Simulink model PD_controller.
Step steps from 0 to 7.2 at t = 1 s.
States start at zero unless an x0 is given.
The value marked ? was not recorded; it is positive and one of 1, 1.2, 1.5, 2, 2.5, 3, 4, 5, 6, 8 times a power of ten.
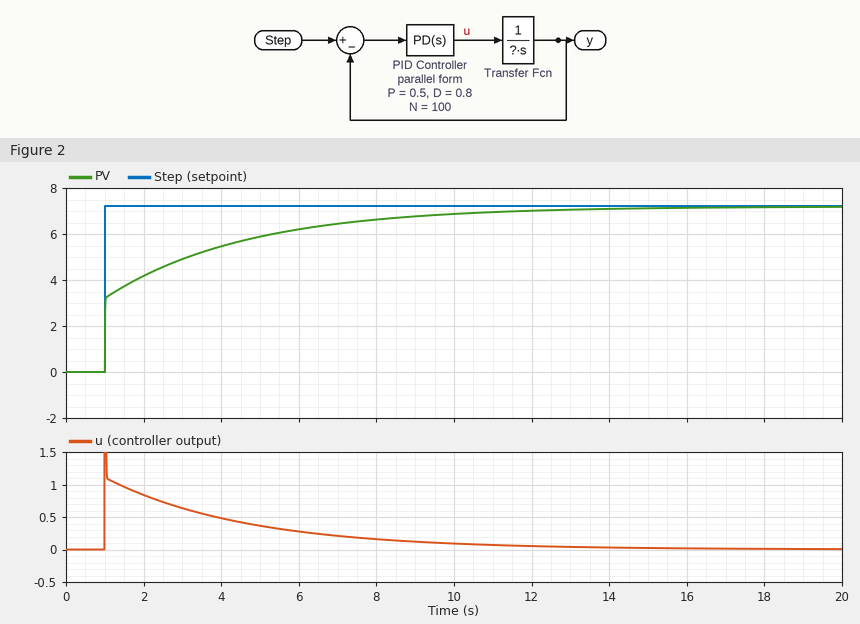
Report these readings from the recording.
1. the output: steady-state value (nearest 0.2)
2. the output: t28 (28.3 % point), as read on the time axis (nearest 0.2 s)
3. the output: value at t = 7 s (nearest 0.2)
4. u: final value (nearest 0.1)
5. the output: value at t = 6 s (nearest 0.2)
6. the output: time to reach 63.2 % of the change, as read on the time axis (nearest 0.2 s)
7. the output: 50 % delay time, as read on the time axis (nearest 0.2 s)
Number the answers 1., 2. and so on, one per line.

1. 7.2
2. 1.0 s
3. 6.4
4. 0.0
5. 6.2
6. 2.4 s
7. 1.4 s
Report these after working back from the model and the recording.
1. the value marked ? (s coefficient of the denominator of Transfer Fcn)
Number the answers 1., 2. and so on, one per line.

1. 1
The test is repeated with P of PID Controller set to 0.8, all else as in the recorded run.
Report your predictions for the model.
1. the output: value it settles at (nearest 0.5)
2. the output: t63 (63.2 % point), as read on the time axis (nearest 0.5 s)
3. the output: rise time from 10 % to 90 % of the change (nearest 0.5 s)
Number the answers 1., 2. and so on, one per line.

1. 7.0
2. 2.0 s
3. 4.0 s
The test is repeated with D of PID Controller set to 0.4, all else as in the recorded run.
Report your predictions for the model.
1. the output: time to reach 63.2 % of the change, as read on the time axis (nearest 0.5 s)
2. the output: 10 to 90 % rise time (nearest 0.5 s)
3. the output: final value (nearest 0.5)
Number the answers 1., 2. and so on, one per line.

1. 3.0 s
2. 5.5 s
3. 7.0
